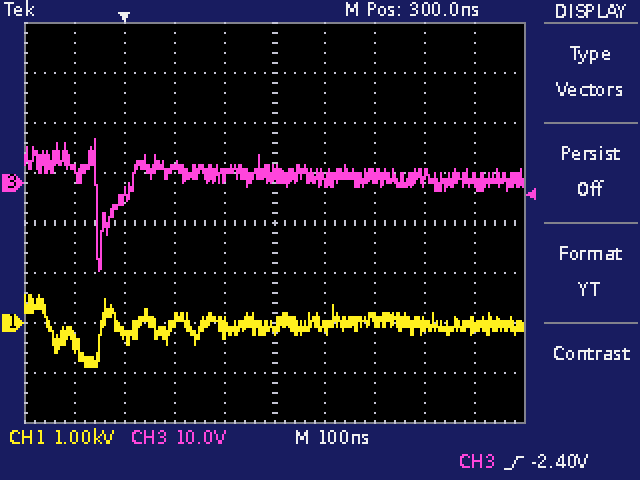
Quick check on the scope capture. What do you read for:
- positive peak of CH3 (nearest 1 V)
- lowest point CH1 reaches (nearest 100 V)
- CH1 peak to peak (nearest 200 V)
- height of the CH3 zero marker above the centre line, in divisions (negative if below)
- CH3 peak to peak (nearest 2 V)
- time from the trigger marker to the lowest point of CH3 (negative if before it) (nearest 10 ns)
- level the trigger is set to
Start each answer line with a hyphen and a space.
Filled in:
- 9 V
- -900 V
- 1.4 kV
- +0.8 div
- 26 V
- -50 ns
- -2.40 V
